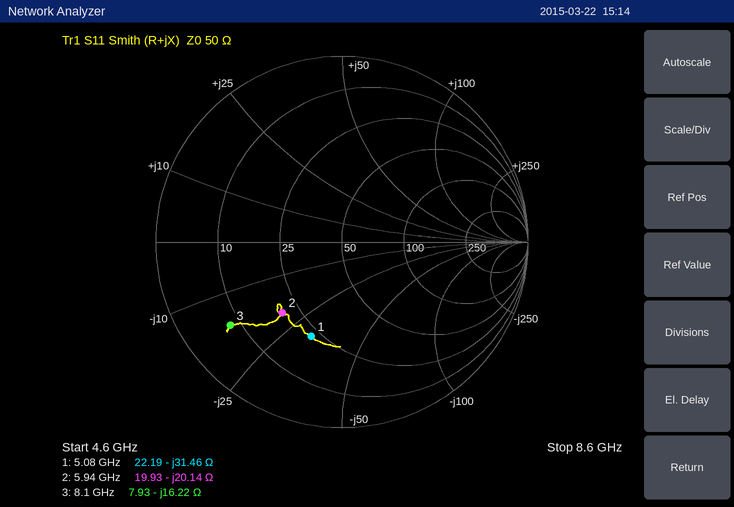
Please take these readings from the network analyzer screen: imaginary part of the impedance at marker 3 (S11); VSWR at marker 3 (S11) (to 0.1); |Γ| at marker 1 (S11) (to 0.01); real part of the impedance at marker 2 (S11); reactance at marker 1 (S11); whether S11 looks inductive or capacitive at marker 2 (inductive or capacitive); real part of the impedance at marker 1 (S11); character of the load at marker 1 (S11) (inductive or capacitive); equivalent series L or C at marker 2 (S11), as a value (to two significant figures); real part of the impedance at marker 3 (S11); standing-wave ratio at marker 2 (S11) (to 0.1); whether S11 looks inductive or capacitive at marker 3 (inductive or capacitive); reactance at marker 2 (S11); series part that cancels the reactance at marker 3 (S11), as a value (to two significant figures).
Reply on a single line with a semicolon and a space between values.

-16.22 Ω; 7.0; 0.53; 19.93 Ω; -31.46 Ω; capacitive; 22.19 Ω; capacitive; 1.3 pF; 7.93 Ω; 3.0; capacitive; -20.14 Ω; 320 pH
